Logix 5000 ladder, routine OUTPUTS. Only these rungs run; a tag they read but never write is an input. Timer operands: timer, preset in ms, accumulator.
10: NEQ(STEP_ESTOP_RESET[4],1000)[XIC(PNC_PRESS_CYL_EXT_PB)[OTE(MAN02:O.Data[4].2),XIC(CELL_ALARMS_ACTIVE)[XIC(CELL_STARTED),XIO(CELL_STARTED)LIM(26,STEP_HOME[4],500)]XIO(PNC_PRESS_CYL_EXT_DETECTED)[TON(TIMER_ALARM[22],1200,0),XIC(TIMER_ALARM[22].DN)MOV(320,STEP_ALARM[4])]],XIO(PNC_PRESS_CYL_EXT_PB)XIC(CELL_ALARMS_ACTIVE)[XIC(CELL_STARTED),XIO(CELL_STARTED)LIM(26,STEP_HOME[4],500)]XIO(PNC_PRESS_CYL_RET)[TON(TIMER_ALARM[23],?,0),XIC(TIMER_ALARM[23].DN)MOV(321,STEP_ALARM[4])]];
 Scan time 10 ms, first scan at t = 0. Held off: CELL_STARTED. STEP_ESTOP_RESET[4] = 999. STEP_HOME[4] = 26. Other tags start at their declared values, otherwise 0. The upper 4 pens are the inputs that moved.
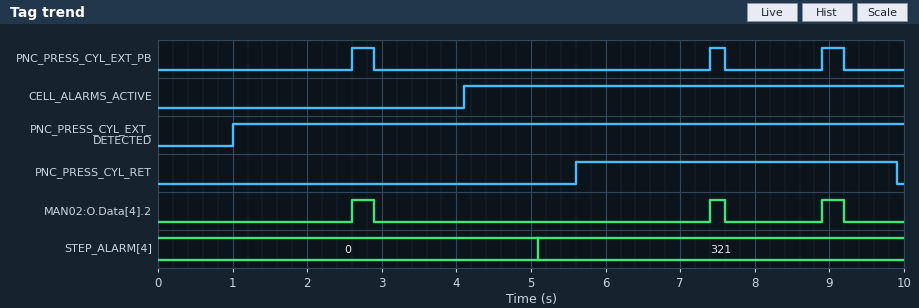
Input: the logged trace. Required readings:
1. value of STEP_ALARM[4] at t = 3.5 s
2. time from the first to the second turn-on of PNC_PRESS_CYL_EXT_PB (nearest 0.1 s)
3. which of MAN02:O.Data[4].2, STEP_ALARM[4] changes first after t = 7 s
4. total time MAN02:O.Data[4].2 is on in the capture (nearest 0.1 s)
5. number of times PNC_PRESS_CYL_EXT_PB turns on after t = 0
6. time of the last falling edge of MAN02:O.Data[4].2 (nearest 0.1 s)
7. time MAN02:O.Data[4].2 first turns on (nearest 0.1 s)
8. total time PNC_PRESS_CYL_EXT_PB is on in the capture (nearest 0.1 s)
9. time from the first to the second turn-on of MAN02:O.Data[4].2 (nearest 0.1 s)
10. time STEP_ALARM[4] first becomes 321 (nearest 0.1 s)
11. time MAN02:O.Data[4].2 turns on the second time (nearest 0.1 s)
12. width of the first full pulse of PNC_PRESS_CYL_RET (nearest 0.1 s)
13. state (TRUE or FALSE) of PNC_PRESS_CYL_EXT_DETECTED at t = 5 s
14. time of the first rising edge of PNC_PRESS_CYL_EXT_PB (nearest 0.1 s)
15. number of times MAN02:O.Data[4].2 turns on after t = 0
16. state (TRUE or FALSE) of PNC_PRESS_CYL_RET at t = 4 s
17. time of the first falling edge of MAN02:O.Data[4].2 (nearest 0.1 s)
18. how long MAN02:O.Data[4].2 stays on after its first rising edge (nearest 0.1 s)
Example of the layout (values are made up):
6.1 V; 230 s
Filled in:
0; 4.8 s; MAN02:O.Data[4].2; 0.8 s; 3; 9.2 s; 2.6 s; 0.8 s; 4.8 s; 5.1 s; 7.4 s; 4.3 s; TRUE; 2.6 s; 3; FALSE; 2.9 s; 0.3 s
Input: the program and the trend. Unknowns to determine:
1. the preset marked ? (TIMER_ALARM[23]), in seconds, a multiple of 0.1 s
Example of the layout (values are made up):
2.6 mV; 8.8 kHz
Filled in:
1.0 s
